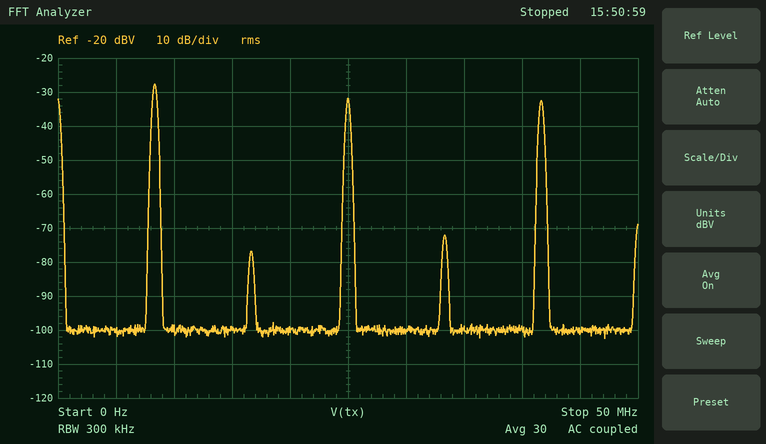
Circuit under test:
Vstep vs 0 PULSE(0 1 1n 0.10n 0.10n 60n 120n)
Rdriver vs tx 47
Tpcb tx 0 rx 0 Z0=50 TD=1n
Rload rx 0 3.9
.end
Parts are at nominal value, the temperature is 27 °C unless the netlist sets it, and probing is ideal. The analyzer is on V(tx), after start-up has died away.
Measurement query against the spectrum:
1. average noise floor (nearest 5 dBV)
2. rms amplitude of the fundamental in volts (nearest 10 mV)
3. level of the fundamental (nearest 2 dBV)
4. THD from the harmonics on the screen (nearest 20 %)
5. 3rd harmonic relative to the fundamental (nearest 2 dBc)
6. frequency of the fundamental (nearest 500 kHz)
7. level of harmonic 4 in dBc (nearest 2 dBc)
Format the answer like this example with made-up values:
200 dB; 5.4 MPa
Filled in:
-100 dBV; 40 mV; -28 dBV; 80 %; -4 dBc; 8.5 MHz; -44 dBc
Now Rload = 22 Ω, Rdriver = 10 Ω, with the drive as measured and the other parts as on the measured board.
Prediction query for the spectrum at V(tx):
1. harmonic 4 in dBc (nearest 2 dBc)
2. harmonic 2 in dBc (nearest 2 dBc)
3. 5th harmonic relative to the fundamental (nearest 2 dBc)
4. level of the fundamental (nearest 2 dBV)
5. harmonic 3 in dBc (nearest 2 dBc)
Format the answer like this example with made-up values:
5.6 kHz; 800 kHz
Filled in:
-52 dBc; -52 dBc; -14 dBc; -10 dBV; -10 dBc
